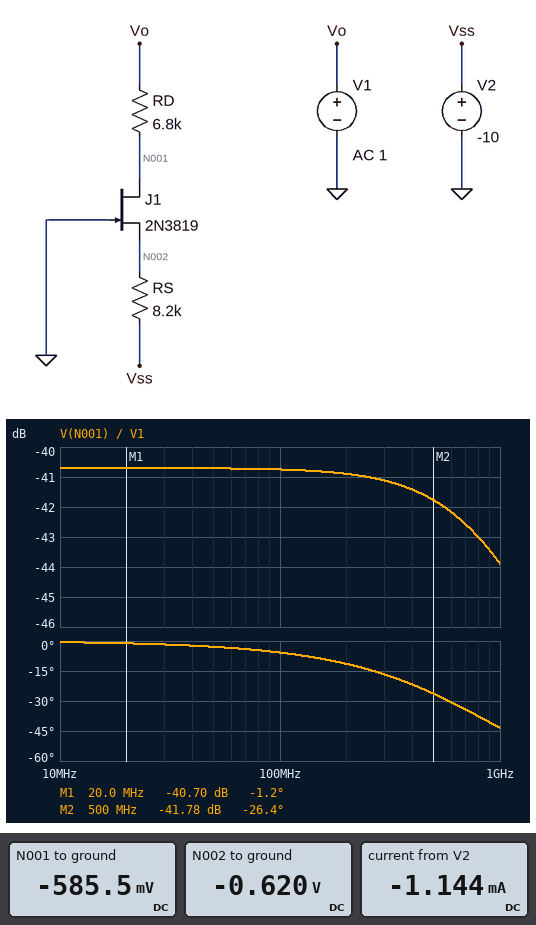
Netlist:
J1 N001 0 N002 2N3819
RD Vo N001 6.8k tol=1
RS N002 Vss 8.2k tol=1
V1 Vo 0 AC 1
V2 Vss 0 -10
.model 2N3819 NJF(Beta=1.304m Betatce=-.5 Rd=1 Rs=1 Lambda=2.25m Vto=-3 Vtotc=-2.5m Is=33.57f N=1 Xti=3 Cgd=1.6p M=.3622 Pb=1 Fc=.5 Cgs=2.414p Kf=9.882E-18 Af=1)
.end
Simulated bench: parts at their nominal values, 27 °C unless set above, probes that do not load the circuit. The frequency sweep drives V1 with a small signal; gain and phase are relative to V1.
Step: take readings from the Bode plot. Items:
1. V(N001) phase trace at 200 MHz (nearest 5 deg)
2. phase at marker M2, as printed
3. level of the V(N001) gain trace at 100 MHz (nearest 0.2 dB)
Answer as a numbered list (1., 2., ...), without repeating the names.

1. -10 deg
2. -26.4 deg
3. -40.8 dB
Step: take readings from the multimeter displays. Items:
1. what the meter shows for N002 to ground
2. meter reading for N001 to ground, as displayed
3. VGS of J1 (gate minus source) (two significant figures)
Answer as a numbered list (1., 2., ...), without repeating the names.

1. -0.620 V
2. -585.5 mV
3. 620 mV
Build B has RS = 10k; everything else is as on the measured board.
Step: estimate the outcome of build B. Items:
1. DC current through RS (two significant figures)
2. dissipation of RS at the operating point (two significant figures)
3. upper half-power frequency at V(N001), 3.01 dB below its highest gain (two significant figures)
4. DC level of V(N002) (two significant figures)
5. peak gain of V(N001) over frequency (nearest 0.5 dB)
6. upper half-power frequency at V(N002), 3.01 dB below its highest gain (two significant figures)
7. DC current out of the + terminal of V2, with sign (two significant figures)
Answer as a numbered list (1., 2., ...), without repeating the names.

1. 940 µA
2. 8.8 mW
3. 840 MHz
4. -610 mV
5. -40.0 dB
6. 670 MHz
7. -940 µA
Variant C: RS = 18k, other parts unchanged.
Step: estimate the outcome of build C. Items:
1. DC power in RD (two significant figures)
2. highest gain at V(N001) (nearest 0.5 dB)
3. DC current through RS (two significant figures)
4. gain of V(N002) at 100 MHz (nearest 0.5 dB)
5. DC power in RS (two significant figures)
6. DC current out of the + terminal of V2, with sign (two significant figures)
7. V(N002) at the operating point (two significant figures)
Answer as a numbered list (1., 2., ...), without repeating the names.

1. 48 µW
2. -37.0 dB
3. 520 µA
4. -44.5 dB
5. 4.9 mW
6. -520 µA
7. -590 mV
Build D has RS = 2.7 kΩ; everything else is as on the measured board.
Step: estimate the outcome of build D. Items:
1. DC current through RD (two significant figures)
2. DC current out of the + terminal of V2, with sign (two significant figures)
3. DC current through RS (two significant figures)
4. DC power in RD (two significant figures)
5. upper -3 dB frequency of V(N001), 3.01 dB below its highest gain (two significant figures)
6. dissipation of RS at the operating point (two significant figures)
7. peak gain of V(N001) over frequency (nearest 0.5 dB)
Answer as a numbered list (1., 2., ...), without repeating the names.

1. 88 µA
2. -3.5 mA
3. 3.5 mA
4. 53 µW
5. 1.5 GHz
6. 32 mW
7. -44.0 dB
